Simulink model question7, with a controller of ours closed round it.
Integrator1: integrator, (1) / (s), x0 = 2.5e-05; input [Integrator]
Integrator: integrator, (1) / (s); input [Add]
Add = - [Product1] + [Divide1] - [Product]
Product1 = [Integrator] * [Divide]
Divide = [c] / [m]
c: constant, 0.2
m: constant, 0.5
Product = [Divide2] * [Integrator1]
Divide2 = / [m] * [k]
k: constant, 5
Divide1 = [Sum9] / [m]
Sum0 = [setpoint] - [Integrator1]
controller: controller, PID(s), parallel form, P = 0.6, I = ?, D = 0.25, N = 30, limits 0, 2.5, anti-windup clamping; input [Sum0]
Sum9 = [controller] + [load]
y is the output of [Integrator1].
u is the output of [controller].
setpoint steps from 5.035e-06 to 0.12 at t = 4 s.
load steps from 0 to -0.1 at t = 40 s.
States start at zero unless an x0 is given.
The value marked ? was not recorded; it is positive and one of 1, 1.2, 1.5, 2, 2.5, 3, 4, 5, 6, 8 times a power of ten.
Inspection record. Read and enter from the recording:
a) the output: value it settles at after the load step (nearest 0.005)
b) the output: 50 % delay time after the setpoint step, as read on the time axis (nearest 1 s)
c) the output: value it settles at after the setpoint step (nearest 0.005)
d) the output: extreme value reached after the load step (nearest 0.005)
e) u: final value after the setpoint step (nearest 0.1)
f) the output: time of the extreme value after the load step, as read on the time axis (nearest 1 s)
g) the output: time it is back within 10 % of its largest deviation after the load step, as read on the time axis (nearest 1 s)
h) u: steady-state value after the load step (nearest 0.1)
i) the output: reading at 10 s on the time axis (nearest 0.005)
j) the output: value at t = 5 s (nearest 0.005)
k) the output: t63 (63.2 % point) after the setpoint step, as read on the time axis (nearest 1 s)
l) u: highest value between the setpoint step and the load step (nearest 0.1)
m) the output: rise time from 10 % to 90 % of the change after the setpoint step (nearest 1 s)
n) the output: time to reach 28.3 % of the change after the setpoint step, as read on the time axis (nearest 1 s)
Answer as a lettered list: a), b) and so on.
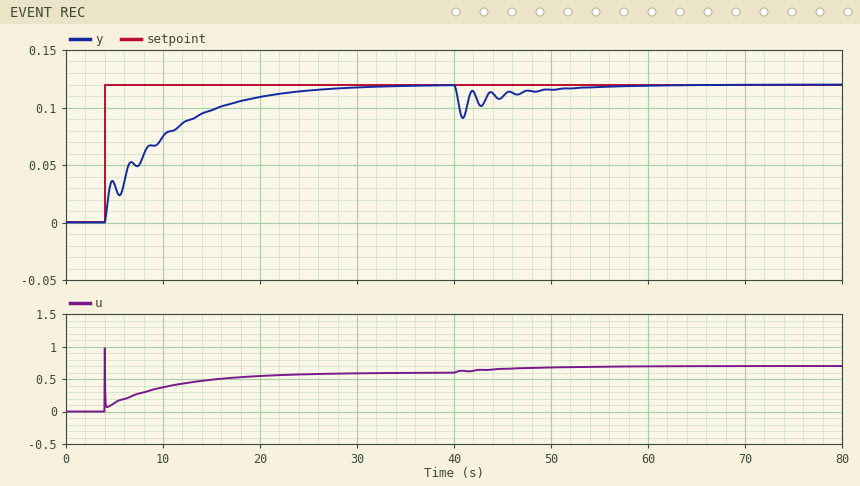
a) 0.120
b) 8 s
c) 0.120
d) 0.090
e) 0.6
f) 41 s
g) 53 s
h) 0.7
i) 0.075
j) 0.035
k) 10 s
l) 1.0
m) 15 s
n) 5 s
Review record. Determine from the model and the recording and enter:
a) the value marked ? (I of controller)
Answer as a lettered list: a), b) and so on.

a) 0.8
